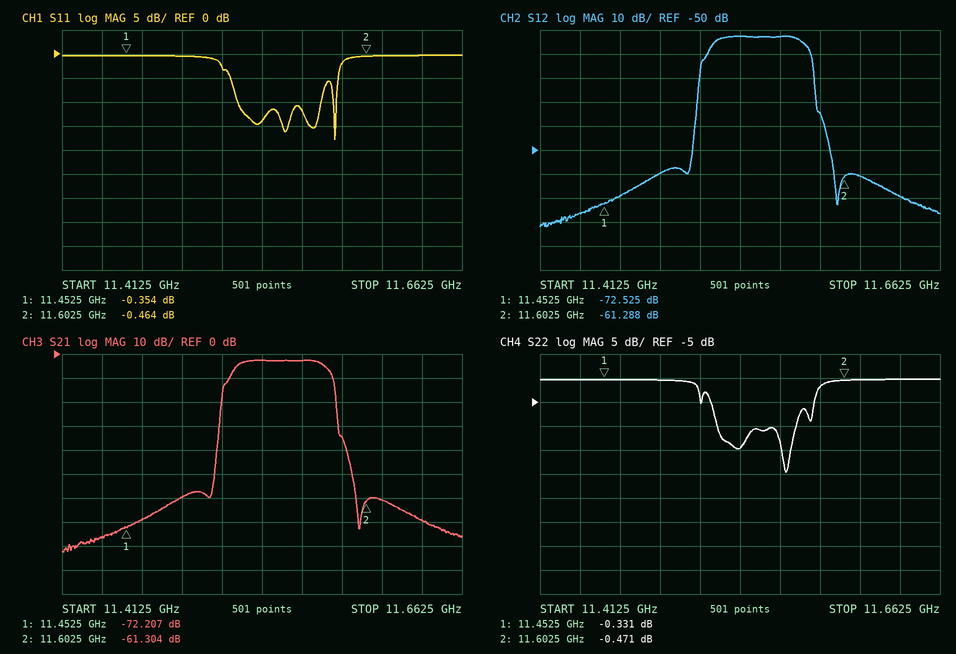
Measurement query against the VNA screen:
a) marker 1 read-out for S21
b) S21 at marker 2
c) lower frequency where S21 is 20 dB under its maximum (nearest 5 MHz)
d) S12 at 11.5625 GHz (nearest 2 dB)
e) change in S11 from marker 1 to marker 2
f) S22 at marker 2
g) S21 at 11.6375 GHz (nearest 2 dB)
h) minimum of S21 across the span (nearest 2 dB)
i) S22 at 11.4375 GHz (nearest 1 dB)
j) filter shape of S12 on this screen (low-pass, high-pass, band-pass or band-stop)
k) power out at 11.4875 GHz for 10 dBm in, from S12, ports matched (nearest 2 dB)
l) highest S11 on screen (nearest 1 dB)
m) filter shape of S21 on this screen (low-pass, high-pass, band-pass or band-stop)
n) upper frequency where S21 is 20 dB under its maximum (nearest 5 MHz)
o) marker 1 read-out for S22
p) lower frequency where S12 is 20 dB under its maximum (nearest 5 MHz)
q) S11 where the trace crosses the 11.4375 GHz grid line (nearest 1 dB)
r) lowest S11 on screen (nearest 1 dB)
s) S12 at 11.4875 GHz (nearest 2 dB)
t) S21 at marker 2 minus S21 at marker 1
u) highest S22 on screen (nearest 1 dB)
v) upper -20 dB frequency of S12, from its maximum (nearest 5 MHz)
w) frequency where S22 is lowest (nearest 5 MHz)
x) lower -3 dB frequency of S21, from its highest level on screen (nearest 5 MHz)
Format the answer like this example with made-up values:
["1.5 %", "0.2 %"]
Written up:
["-72.207 dB", "-61.304 dB", "11.510 GHz", "-2 dB", "-0.110 dB", "-0.471 dB", "-70 dB", "-82 dB", "0 dB", "band-pass", "-50 dBm", "0 dB", "band-pass", "11.585 GHz", "-0.331 dB", "11.510 GHz", "0 dB", "-18 dB", "-60 dB", "10.903 dB", "0 dB", "11.585 GHz", "11.565 GHz", "11.520 GHz"]
